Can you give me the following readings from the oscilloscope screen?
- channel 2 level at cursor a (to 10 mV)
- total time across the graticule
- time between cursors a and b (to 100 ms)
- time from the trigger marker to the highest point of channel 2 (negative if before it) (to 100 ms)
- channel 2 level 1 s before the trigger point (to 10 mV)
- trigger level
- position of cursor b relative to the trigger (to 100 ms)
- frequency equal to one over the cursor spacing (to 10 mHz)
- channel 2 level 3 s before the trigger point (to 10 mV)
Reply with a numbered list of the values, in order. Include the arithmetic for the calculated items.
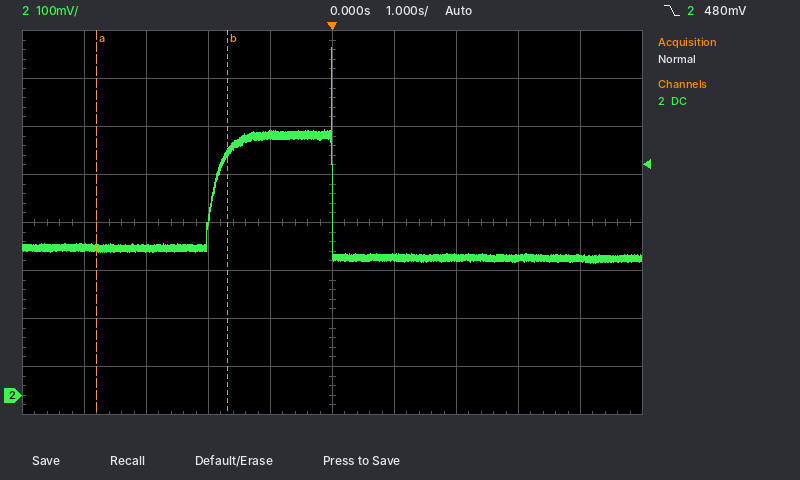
1. 310 mV
2. 10 s
3. 2.1 s
4. 0.0 s
5. 540 mV
6. 480 mV
7. -1.7 s
8. 1 / 2.1 s ≈ 480 mHz
9. 310 mV
